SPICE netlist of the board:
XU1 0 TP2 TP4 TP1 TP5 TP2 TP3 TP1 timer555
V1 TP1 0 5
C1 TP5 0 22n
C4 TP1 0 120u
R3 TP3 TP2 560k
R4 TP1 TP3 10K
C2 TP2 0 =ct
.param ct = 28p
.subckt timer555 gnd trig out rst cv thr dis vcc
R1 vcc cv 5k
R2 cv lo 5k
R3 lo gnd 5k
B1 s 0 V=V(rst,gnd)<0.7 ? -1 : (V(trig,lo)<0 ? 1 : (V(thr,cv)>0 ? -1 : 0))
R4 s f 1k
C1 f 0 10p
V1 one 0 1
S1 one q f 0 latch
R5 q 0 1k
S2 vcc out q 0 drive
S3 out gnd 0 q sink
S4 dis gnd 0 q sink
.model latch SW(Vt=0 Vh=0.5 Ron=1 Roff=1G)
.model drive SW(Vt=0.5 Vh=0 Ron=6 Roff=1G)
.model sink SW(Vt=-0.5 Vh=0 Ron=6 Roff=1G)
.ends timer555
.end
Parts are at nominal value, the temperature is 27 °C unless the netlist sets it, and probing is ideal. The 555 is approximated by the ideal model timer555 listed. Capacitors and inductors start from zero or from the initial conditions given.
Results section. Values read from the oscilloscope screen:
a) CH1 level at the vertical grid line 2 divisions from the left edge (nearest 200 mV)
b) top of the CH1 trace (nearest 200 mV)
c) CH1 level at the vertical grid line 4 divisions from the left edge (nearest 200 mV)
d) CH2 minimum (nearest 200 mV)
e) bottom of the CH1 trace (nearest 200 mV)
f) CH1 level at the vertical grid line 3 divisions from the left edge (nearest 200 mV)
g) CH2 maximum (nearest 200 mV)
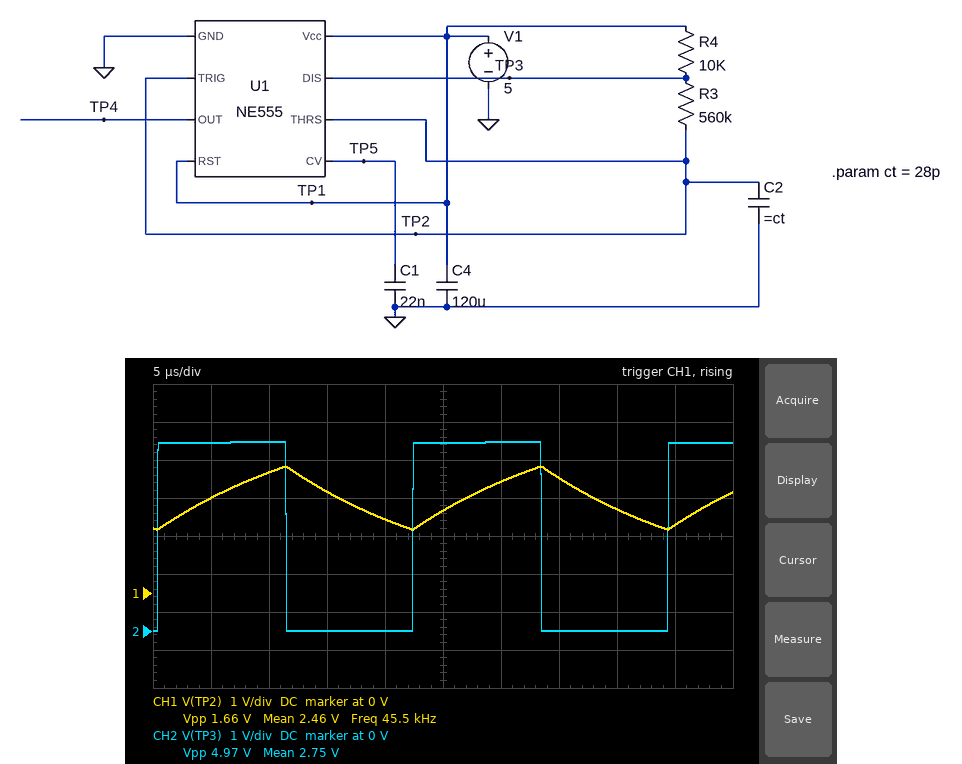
3.2 V
3.4 V
2.0 V
0 V
1.6 V
2.6 V
5.0 V
